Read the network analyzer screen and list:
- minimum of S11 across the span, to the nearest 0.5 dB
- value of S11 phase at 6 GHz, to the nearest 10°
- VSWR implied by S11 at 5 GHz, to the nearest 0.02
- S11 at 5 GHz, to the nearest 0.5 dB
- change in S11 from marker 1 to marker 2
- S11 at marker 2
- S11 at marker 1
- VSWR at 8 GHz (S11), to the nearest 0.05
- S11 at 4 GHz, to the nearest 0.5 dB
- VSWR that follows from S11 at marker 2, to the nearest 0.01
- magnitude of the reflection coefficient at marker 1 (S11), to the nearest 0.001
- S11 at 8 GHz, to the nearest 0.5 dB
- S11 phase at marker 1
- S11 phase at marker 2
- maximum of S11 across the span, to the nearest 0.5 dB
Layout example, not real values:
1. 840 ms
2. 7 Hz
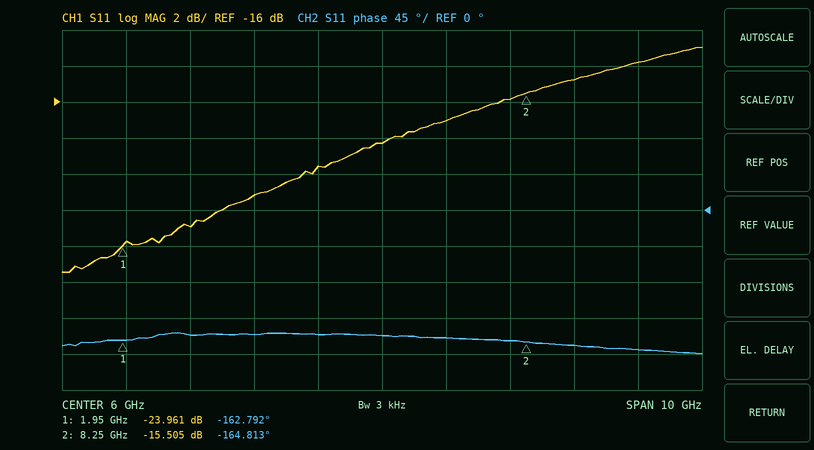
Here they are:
1. -25.5 dB
2. -160°
3. 1.24
4. -19.5 dB
5. 8.456 dB
6. -15.505 dB
7. -23.961 dB
8. 1.40
9. -21.0 dB
10. 1.40
11. 0.063
12. -16.0 dB
13. -162.792°
14. -164.813°
15. -13.0 dB
